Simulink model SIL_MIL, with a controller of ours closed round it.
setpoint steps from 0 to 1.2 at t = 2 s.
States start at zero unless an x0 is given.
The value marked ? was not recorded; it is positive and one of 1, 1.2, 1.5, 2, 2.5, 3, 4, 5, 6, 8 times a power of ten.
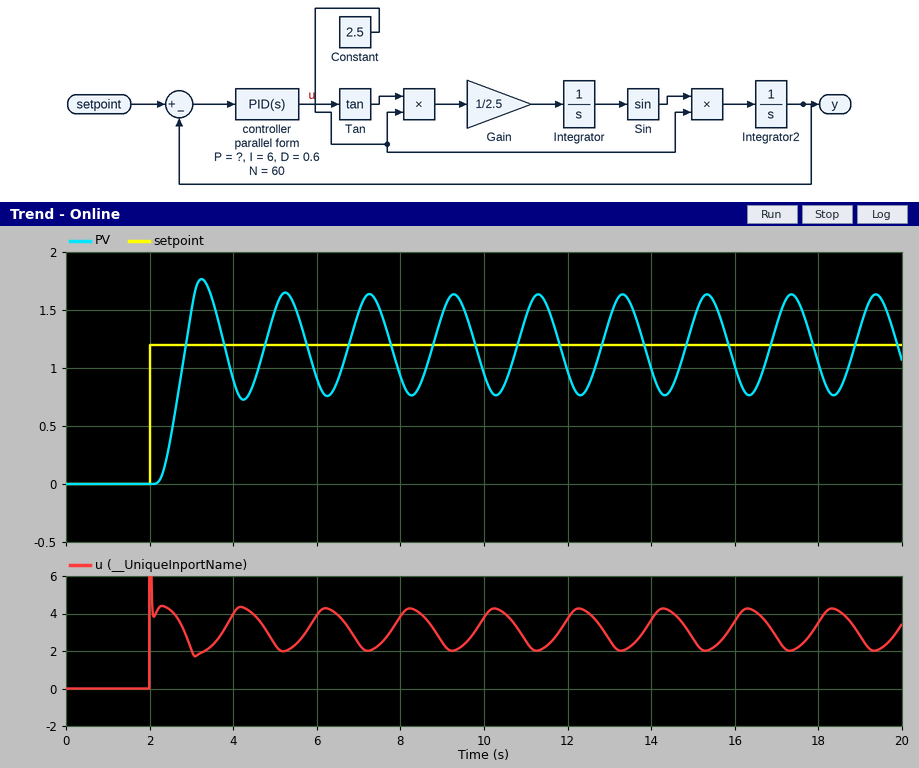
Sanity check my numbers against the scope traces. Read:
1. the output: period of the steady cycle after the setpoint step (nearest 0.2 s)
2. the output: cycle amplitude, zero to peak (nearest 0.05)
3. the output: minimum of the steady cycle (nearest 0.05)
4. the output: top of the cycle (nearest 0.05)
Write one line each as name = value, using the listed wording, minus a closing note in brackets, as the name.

the output: period of the steady cycle after the setpoint step = 2.0 s
the output: cycle amplitude, zero to peak = 0.45
the output: minimum of the steady cycle = 0.75
the output: top of the cycle = 1.65
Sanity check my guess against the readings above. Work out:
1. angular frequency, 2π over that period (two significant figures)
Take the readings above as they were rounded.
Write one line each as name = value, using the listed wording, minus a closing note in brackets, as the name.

angular frequency, 2π over that period = 3.1 rad/s
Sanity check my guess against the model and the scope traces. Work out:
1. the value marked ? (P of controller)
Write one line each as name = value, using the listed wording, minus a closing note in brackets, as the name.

the value marked ? = 2.5
